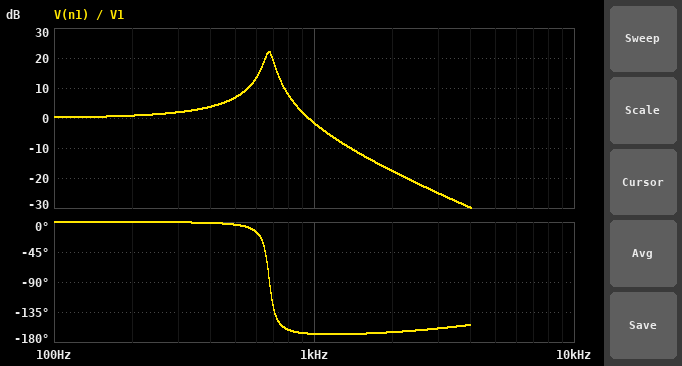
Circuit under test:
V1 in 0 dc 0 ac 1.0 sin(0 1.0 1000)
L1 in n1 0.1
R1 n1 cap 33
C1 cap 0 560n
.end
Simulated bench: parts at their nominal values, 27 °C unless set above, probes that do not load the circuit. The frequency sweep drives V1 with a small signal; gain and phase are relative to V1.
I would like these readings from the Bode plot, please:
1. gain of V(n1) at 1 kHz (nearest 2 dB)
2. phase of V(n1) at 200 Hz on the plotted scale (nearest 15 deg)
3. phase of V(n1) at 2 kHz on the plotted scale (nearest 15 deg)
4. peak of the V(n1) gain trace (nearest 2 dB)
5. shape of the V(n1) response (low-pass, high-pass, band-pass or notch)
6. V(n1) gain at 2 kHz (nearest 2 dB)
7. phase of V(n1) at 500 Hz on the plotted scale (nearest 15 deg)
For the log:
-2 dB
0 deg
-165 deg
22 dB
low-pass
-18 dB
0 deg
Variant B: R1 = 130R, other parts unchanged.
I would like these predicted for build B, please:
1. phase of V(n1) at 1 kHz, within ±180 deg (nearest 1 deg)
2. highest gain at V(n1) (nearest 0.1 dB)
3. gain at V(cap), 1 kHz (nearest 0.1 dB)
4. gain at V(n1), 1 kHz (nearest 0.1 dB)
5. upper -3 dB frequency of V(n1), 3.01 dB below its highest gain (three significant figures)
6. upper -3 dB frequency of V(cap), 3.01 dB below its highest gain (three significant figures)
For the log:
-135 deg
10.7 dB
-2.2 dB
-1.4 dB
756 Hz
754 Hz
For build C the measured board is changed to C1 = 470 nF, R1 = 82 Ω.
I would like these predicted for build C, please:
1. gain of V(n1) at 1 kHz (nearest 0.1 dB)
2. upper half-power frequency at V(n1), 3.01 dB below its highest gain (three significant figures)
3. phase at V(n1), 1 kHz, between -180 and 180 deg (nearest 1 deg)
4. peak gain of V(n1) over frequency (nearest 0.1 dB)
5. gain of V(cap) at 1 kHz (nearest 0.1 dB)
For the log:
1.3 dB
791 Hz
-151 deg
15.2 dB
1.0 dB
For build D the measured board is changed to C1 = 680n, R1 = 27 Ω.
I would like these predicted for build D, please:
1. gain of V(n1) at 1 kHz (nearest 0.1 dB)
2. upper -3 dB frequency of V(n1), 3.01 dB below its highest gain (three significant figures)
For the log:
-4.5 dB
631 Hz
